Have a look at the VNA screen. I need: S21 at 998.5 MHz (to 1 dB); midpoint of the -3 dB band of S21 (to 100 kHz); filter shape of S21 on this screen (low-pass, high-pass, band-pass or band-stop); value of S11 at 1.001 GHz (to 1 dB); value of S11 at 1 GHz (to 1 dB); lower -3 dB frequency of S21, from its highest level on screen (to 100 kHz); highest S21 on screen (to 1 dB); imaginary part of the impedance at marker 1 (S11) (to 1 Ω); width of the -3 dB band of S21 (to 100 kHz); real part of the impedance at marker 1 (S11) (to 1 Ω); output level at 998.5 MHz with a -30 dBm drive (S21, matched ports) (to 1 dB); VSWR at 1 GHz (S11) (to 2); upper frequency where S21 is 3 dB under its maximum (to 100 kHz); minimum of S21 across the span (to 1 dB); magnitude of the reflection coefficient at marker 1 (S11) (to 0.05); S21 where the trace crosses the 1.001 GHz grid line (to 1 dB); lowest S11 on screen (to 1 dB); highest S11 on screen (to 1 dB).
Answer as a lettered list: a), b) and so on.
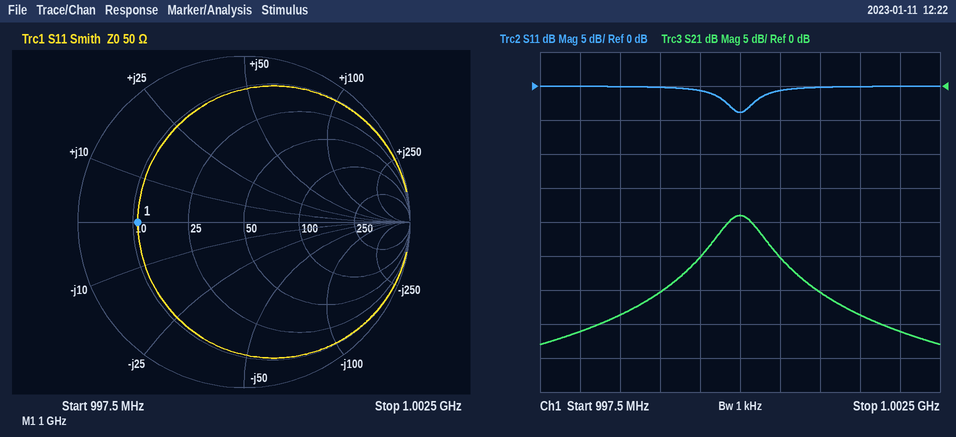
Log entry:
a) -34 dB
b) 1.0000 GHz
c) band-pass
d) 0 dB
e) -4 dB
f) 999.7 MHz
g) -19 dB
h) 0 Ω
i) 600 kHz
j) 11 Ω
k) -64 dBm
l) 4
m) 1.0003 GHz
n) -38 dB
o) 0.65
p) -30 dB
q) -4 dB
r) 0 dB
